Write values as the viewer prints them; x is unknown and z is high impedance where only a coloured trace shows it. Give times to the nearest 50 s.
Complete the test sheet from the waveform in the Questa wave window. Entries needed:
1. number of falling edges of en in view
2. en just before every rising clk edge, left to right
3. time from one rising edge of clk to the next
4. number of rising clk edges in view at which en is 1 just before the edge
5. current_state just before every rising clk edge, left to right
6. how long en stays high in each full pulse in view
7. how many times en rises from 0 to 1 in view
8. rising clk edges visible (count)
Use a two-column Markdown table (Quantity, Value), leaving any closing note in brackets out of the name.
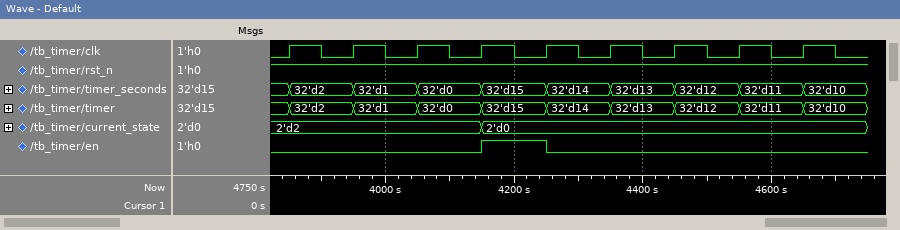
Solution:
| Quantity | Value |
|---|---|
| number of falling edges of en in view | 1 |
| en just before every rising clk edge, left to right | 0 0 0 0 1 0 0 0 0 |
| time from one rising edge of clk to the next | 100 s |
| number of rising clk edges in view at which en is 1 just before the edge | 1 |
| current_state just before every rising clk edge, left to right | 2'd2, 2'd2, 2'd2, 2'd2, 2'd0, 2'd0, 2'd0, 2'd0, 2'd0 |
| how long en stays high in each full pulse in view | 100 s |
| how many times en rises from 0 to 1 in view | 1 |
| rising clk edges visible | 9 |
